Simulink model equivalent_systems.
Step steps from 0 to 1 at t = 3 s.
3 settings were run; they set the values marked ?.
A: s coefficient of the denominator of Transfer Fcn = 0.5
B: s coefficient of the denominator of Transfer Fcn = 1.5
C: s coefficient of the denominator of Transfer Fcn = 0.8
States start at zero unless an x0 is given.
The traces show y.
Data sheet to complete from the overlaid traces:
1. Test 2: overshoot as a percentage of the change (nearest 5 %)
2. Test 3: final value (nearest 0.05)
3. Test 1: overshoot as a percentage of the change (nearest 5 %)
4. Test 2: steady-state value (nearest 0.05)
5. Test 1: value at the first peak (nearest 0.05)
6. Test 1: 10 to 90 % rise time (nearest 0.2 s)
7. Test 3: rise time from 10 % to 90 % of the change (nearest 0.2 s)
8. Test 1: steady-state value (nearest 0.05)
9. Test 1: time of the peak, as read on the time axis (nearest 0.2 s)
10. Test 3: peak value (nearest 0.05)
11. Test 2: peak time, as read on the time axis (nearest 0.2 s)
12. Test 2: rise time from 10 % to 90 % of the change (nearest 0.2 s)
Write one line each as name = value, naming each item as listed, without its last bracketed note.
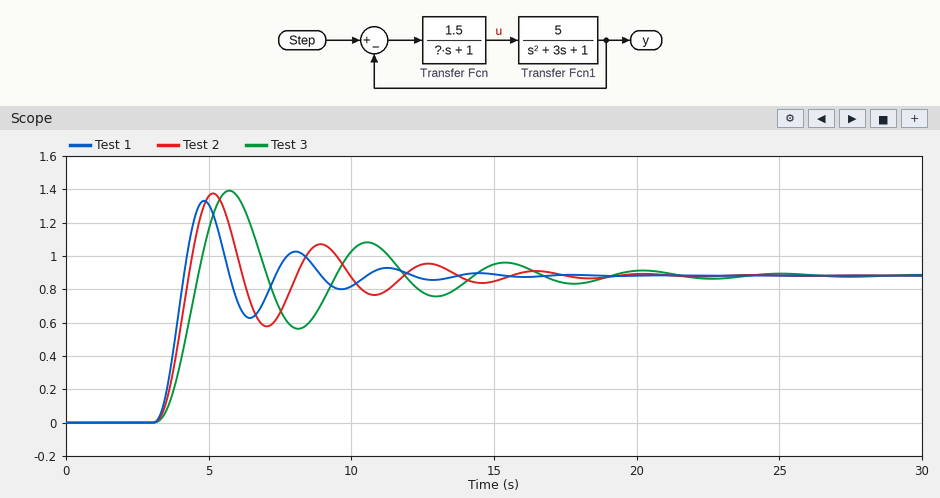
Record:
Test 2: overshoot as a percentage of the change = 55 %
Test 3: final value = 0.90
Test 1: overshoot as a percentage of the change = 50 %
Test 2: steady-state value = 0.90
Test 1: value at the first peak = 1.35
Test 1: 10 to 90 % rise time = 0.6 s
Test 3: rise time from 10 % to 90 % of the change = 1.0 s
Test 1: steady-state value = 0.90
Test 1: time of the peak, as read on the time axis = 4.8 s
Test 3: peak value = 1.40
Test 2: peak time, as read on the time axis = 5.2 s
Test 2: rise time from 10 % to 90 % of the change = 0.8 s
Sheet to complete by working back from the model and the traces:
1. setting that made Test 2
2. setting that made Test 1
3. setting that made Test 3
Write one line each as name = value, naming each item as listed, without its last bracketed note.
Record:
setting that made Test 2 = C
setting that made Test 1 = A
setting that made Test 3 = B
